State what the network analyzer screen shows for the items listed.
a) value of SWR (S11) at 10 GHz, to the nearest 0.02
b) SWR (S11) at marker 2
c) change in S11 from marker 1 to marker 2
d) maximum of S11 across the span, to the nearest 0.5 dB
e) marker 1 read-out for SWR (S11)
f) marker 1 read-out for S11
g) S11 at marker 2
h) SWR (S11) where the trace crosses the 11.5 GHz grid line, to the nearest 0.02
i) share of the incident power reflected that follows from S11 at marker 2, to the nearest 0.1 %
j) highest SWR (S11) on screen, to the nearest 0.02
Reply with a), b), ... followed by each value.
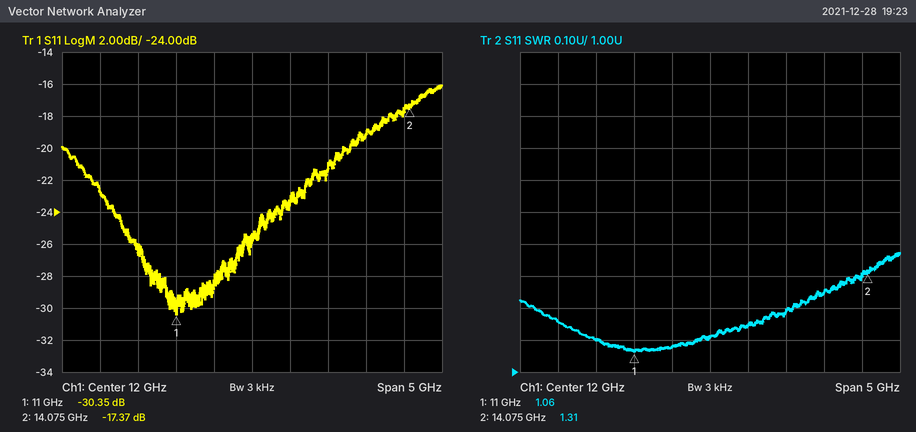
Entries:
a) 1.16
b) 1.31
c) 12.98 dB
d) -16.0 dB
e) 1.06
f) -30.35 dB
g) -17.37 dB
h) 1.08
i) 1.8 %
j) 1.38
